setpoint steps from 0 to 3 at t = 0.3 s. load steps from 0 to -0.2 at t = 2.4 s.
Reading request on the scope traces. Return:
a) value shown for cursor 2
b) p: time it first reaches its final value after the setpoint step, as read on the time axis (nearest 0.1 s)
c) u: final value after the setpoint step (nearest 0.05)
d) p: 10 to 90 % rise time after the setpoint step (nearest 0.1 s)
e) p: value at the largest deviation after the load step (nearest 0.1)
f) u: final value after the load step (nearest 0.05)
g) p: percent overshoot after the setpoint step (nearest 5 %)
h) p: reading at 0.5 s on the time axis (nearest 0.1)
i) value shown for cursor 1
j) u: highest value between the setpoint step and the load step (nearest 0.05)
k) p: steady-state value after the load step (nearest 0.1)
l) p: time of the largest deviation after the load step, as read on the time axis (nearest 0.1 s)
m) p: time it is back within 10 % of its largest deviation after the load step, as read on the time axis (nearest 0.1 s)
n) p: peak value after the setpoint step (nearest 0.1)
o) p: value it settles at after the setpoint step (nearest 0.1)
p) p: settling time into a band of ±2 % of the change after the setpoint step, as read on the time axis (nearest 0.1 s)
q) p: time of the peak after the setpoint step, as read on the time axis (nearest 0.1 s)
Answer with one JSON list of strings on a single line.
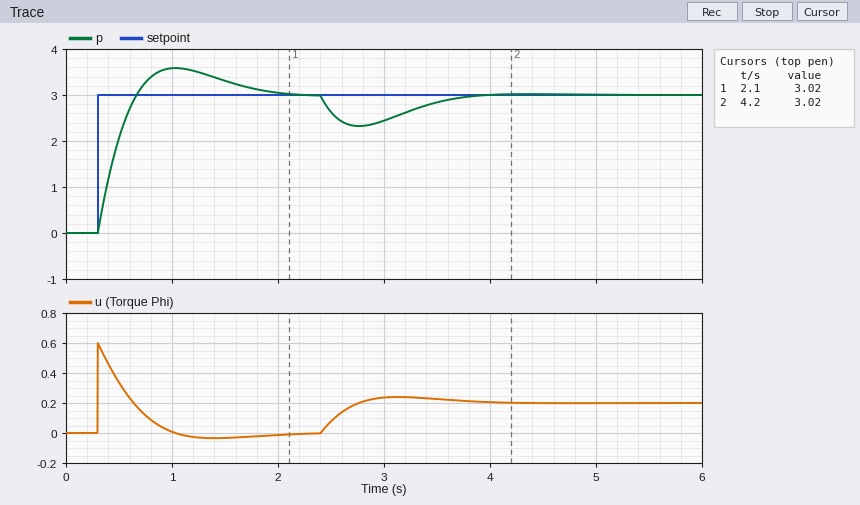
["3.02", "0.7 s", "0.00", "0.3 s", "2.3", "0.20", "20 %", "2.1", "3.02", "0.60", "3.0", "2.8 s", "3.7 s", "3.6", "3.0", "2.0 s", "1.0 s"]
